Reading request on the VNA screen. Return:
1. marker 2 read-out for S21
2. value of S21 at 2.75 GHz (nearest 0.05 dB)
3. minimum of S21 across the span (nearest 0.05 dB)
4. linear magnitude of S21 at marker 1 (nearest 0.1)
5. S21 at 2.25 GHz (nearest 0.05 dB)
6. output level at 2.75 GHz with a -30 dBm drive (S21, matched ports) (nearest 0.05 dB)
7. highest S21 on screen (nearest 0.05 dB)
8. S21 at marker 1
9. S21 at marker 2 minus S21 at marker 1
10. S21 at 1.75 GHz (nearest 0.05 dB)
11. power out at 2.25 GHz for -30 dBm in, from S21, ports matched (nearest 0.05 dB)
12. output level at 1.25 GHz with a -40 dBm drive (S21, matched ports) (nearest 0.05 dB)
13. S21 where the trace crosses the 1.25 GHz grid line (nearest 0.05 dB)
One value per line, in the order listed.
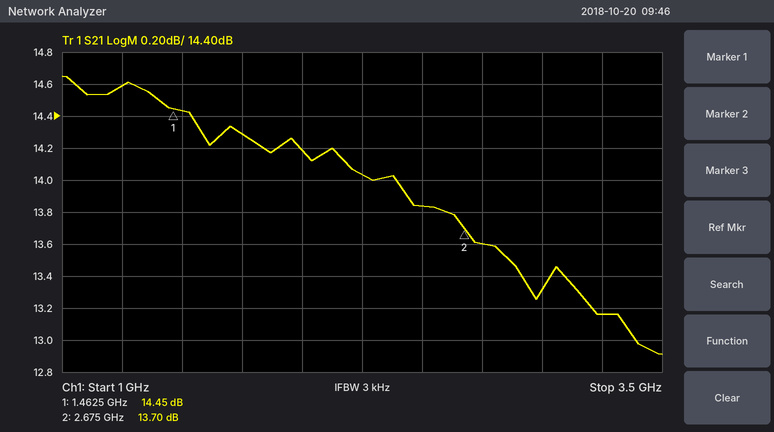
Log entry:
13.70 dB
13.60 dB
12.90 dB
5.3
14.05 dB
-16.40 dBm
14.65 dB
14.45 dB
-0.75 dB
14.30 dB
-15.95 dBm
-25.40 dBm
14.60 dB
